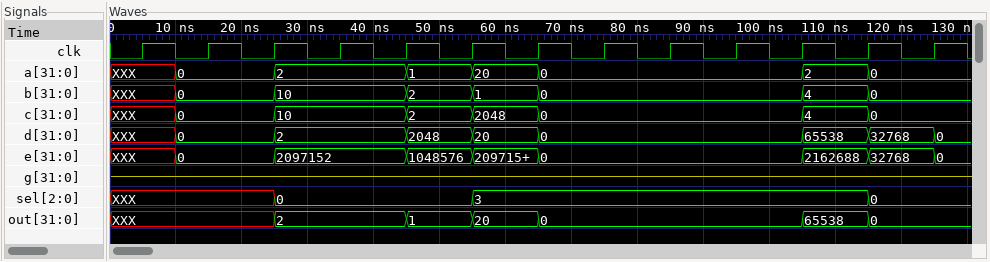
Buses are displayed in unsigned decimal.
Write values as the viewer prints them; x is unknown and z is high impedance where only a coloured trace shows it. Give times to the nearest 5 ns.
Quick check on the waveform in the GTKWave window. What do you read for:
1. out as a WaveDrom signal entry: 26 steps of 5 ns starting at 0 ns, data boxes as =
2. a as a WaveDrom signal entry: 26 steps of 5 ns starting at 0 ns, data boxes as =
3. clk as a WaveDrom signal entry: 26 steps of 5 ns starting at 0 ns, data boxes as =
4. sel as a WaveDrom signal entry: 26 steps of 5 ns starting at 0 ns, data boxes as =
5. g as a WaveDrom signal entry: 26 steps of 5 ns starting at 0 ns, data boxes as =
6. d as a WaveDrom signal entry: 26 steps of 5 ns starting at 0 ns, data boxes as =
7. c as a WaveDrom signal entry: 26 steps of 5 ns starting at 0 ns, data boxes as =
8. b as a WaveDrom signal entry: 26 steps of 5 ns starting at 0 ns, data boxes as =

{name: 'out', wave: 'x....=...=.=.=.......=.=..', data: '2 1 20 0 65538 0'}
{name: 'a', wave: 'x.=..=...=.=.=.......=.=..', data: '0 2 1 20 0 2 0'}
{name: 'clk', wave: '01010101010101010101010101'}
{name: 'sel', wave: 'x....=.....=...........=..', data: '0 3 0'}
{name: 'g', wave: 'z.........................'}
{name: 'd', wave: 'x.=..=...=.=.=.......=.=.=', data: '0 2 2048 20 0 65538 32768 0'}
{name: 'c', wave: 'x.=..=...=.=.=.......=.=..', data: '0 10 2 2048 0 4 0'}
{name: 'b', wave: 'x.=..=...=.=.=.......=.=..', data: '0 10 2 1 0 4 0'}
